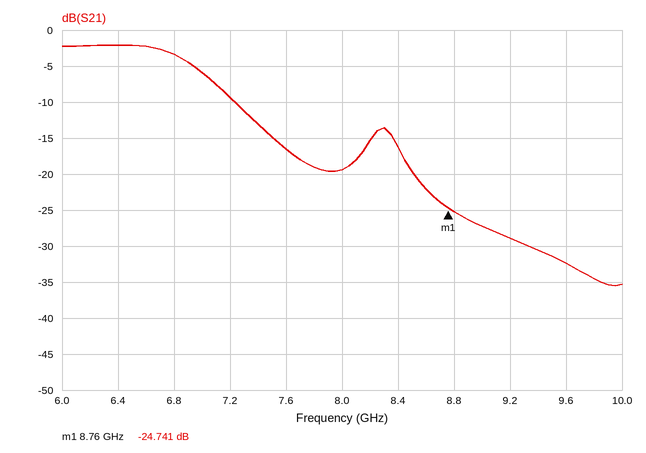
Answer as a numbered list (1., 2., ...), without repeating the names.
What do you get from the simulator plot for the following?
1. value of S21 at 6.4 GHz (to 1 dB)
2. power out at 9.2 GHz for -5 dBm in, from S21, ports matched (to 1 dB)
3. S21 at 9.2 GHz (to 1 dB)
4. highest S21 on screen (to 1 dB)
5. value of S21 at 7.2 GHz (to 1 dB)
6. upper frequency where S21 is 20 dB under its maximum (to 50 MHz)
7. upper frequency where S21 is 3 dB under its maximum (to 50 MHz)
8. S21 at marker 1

1. -2 dB
2. -34 dBm
3. -29 dB
4. -2 dB
5. -9 dB
6. 8.60 GHz
7. 6.95 GHz
8. -24.741 dB
